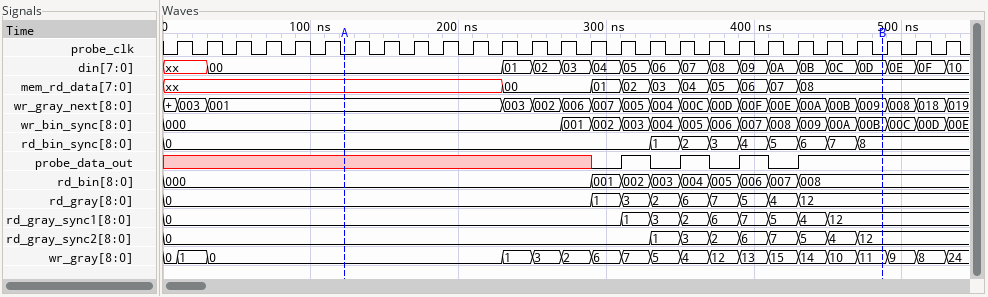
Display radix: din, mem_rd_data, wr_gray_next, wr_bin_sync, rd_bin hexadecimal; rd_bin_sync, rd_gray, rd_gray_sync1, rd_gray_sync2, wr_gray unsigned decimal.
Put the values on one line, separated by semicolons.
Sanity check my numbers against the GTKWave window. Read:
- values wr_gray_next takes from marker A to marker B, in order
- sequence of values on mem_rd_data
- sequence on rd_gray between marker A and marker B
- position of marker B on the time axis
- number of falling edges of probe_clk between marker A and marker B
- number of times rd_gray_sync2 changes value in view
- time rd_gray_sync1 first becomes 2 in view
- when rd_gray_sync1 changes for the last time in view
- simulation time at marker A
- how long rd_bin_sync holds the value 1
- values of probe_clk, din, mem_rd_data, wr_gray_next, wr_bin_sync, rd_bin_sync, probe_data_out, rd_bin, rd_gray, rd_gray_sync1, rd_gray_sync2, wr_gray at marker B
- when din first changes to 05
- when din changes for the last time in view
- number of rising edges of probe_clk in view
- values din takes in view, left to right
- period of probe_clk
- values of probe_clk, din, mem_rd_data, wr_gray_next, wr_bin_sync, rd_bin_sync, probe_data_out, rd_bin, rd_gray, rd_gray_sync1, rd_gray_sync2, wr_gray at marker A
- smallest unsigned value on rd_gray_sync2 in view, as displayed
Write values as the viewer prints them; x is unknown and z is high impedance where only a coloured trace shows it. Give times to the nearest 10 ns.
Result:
001, 003, 002, 006, 007, 005, 004, 00C, 00D, 00F, 00E, 00A, 00B, 009; xx, 00, 01, 02, 03, 04, 05, 06, 07, 08; 0, 1, 3, 2, 6, 7, 5, 4, 12; 490 ns; 18; 8; 350 ns; 450 ns; 120 ns; 20 ns; probe_clk=0, din=0D, mem_rd_data=08, wr_gray_next=009, wr_bin_sync=00B, rd_bin_sync=8, probe_data_out=1, rd_bin=008, rd_gray=12, rd_gray_sync1=12, rd_gray_sync2=12, wr_gray=11; 310 ns; 530 ns; 27; xx, 00, 01, 02, 03, 04, 05, 06, 07, 08, 09, 0A, 0B, 0C, 0D, 0E, 0F, 10; 20 ns; probe_clk=0, din=00, mem_rd_data=xx, wr_gray_next=001, wr_bin_sync=000, rd_bin_sync=0, probe_data_out=x, rd_bin=000, rd_gray=0, rd_gray_sync1=0, rd_gray_sync2=0, wr_gray=0; 0
